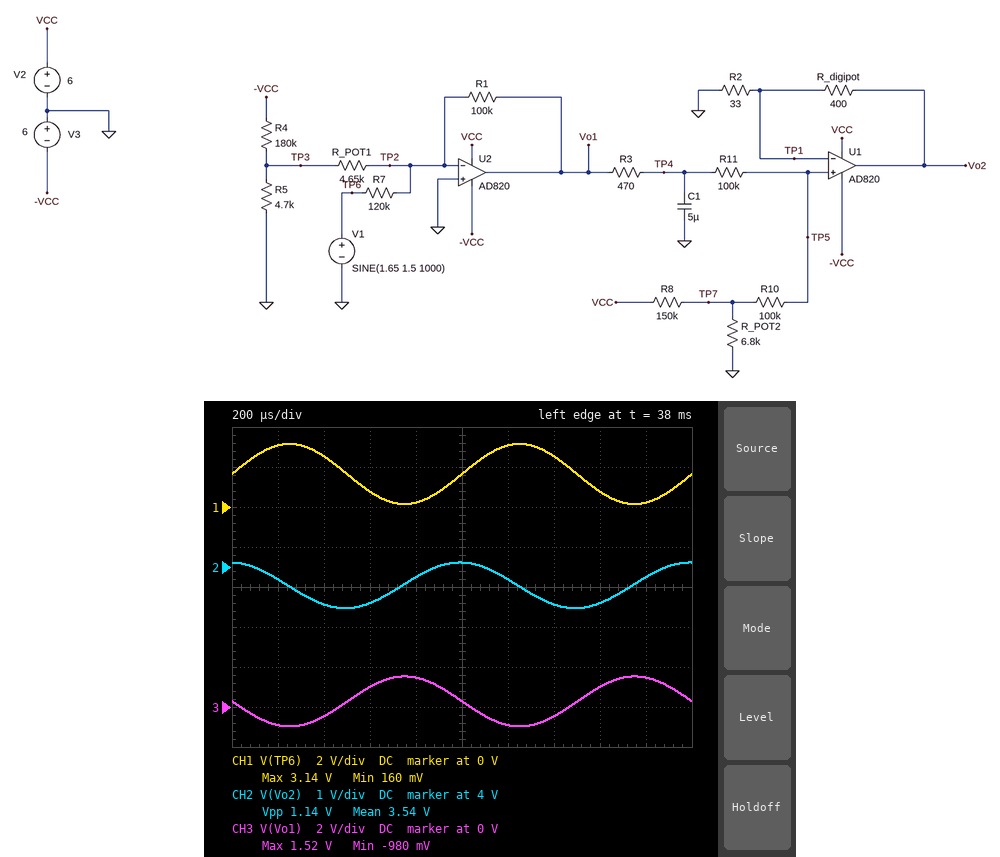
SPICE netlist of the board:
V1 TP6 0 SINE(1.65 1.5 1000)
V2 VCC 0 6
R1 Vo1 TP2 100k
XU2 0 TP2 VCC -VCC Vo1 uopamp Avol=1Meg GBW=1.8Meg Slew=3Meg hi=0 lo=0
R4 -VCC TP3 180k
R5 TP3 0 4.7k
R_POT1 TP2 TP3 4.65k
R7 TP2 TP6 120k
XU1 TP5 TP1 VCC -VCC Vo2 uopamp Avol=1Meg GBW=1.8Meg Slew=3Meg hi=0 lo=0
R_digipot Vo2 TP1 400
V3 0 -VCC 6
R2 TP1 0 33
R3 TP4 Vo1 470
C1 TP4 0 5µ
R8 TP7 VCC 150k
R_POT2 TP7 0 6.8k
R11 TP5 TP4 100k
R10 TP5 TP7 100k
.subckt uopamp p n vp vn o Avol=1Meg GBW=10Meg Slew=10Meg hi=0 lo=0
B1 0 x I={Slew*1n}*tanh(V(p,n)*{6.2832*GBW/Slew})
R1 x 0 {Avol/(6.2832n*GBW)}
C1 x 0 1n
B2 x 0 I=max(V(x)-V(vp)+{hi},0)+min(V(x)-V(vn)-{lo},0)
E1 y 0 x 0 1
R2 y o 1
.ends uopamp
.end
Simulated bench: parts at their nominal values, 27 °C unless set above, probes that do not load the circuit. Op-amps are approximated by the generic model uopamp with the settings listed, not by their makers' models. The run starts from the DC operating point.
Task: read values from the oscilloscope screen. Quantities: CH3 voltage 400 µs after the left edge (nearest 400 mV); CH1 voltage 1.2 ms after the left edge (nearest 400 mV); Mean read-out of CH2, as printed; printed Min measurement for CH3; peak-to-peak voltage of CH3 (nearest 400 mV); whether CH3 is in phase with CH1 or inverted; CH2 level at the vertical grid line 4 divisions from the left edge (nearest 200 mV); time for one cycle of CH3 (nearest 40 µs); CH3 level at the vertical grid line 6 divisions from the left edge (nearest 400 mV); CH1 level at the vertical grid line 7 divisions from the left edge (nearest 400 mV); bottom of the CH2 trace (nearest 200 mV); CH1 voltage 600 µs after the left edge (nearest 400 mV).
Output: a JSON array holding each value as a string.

["-400 mV", "3.2 V", "3.54 V", "-980 mV", "2.4 V", "inverted", "3.8 V", "1.00 ms", "-800 mV", "2.4 V", "3.0 V", "800 mV"]
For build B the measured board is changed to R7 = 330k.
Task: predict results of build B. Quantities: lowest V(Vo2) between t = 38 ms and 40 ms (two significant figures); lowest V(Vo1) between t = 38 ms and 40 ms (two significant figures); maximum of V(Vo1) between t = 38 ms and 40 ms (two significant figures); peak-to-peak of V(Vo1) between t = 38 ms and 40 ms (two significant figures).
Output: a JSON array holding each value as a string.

["6.0 V", "700 mV", "1.6 V", "910 mV"]
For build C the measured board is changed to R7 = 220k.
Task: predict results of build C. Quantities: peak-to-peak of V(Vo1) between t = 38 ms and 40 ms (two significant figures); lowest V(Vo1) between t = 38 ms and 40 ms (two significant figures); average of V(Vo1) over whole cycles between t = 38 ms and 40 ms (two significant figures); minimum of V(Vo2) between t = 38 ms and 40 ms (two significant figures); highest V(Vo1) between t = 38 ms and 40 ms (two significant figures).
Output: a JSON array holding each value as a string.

["1.4 V", "220 mV", "900 mV", "6.0 V", "1.6 V"]
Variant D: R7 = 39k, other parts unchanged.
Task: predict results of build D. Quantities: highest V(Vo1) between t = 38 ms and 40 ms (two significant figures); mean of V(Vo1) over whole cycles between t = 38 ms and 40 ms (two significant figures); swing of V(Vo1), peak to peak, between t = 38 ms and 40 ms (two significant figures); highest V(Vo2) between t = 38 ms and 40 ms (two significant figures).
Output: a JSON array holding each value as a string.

["1.3 V", "-2.5 V", "7.3 V", "-6.0 V"]
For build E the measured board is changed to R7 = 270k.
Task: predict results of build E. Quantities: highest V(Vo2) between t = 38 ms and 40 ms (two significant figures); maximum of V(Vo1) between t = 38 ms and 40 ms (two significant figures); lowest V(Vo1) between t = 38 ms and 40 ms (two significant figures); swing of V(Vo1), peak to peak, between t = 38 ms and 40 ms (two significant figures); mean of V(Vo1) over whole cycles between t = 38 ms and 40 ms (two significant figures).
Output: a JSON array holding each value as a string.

["6.0 V", "1.6 V", "490 mV", "1.1 V", "1.0 V"]
